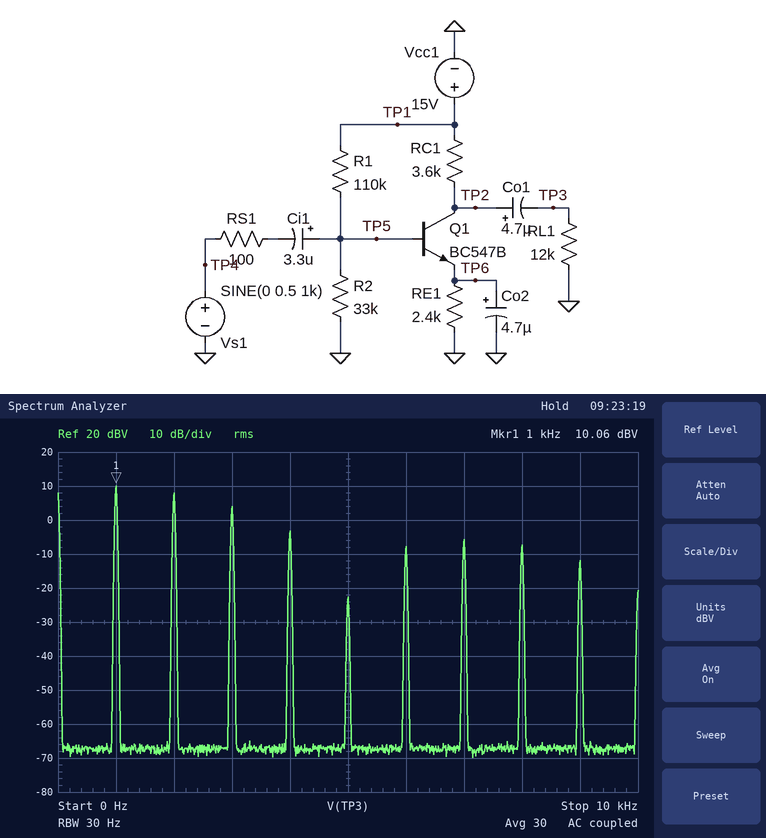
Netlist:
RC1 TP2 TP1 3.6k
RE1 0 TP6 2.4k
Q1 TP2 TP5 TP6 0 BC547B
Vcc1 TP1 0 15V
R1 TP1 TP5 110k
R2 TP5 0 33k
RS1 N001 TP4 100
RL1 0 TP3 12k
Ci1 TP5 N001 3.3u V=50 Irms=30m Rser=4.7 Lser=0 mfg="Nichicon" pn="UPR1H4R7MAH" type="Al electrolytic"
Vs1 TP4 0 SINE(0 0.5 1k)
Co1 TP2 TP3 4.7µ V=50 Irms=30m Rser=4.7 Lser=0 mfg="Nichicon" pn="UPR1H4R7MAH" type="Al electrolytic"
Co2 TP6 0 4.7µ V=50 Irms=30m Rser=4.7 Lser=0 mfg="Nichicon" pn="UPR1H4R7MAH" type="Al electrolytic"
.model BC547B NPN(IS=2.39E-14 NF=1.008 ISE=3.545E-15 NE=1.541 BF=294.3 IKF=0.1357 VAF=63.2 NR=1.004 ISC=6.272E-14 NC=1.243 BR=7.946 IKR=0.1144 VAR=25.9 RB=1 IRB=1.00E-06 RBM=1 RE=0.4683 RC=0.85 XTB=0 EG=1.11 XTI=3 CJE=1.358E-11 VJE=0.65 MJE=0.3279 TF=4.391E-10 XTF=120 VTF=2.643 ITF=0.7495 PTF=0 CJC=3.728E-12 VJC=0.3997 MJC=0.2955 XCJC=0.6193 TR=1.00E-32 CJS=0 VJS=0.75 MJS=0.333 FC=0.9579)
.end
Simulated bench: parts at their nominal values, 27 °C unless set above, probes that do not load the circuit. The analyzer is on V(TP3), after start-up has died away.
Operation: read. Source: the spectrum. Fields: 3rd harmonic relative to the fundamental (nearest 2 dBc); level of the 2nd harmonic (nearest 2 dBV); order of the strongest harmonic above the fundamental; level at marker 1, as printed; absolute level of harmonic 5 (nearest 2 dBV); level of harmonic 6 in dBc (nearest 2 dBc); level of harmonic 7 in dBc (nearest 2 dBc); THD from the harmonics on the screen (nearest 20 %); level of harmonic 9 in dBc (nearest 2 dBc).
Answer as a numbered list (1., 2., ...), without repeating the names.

1. -6 dBc
2. 8 dBV
3. 2
4. 10.06 dBV
5. -22 dBV
6. -18 dBc
7. -16 dBc
8. 100 %
9. -22 dBc
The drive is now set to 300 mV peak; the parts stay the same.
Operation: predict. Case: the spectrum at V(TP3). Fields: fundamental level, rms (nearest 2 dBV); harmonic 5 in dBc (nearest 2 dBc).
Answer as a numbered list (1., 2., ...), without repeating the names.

1. 10 dBV
2. -22 dBc
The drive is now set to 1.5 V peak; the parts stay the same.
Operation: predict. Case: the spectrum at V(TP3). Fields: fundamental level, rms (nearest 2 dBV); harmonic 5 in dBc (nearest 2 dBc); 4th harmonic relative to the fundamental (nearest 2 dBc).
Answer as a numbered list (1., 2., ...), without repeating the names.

1. 8 dBV
2. -12 dBc
3. -6 dBc
